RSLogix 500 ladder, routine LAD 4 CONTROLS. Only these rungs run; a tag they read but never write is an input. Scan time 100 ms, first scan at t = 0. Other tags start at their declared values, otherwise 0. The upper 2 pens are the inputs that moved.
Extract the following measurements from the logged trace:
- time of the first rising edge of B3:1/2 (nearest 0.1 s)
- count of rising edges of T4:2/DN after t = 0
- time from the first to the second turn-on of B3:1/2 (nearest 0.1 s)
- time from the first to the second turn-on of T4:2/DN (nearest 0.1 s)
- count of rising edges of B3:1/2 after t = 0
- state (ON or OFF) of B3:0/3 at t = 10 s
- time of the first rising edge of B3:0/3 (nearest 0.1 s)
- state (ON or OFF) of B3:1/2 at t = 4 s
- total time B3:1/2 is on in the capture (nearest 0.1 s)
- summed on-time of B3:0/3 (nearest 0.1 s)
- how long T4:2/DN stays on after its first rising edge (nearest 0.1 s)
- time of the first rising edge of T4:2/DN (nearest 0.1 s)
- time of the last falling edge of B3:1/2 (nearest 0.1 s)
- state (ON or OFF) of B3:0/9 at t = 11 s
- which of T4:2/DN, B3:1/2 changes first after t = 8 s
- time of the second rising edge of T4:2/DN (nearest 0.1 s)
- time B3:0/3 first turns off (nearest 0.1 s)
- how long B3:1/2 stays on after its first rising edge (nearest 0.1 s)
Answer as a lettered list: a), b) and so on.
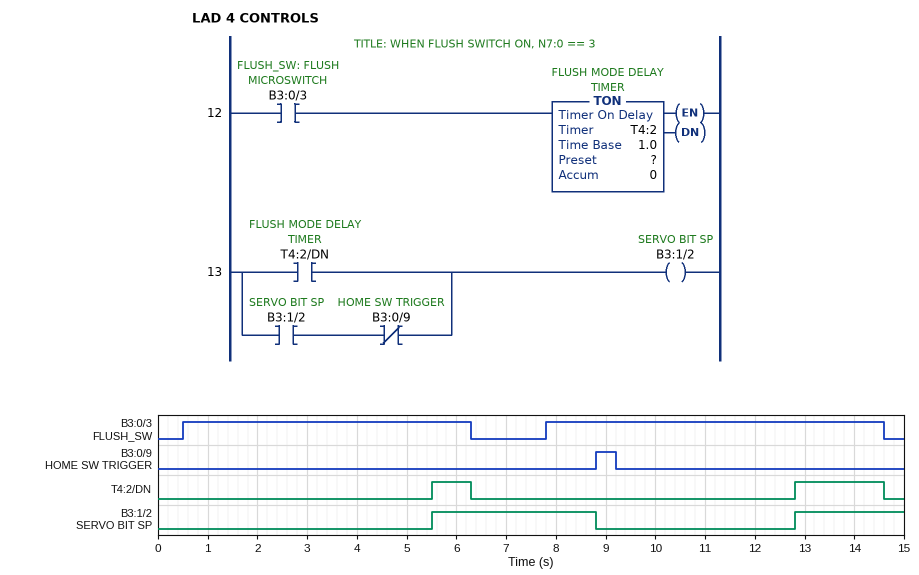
a) 5.5 s
b) 2
c) 7.3 s
d) 7.3 s
e) 2
f) ON
g) 0.5 s
h) OFF
i) 5.5 s
j) 12.6 s
k) 0.8 s
l) 5.5 s
m) 8.8 s
n) OFF
o) B3:1/2
p) 12.8 s
q) 6.3 s
r) 3.3 s
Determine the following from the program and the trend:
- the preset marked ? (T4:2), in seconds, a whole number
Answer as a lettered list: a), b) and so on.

a) 5 s
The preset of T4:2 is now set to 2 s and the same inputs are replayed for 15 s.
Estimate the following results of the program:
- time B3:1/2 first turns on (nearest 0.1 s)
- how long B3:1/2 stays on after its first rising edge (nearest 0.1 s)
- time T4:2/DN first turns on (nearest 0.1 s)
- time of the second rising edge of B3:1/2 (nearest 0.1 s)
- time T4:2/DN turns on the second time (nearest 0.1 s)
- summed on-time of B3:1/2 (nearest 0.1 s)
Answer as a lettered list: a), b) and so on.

a) 2.5 s
b) 6.3 s
c) 2.5 s
d) 9.8 s
e) 9.8 s
f) 11.5 s
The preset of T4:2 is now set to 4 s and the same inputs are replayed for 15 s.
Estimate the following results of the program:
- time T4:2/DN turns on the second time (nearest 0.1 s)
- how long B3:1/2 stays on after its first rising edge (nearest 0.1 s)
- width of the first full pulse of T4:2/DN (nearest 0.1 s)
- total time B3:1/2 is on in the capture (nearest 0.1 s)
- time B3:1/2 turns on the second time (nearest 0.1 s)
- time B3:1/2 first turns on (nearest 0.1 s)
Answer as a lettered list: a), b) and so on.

a) 11.8 s
b) 4.3 s
c) 1.8 s
d) 7.5 s
e) 11.8 s
f) 4.5 s
